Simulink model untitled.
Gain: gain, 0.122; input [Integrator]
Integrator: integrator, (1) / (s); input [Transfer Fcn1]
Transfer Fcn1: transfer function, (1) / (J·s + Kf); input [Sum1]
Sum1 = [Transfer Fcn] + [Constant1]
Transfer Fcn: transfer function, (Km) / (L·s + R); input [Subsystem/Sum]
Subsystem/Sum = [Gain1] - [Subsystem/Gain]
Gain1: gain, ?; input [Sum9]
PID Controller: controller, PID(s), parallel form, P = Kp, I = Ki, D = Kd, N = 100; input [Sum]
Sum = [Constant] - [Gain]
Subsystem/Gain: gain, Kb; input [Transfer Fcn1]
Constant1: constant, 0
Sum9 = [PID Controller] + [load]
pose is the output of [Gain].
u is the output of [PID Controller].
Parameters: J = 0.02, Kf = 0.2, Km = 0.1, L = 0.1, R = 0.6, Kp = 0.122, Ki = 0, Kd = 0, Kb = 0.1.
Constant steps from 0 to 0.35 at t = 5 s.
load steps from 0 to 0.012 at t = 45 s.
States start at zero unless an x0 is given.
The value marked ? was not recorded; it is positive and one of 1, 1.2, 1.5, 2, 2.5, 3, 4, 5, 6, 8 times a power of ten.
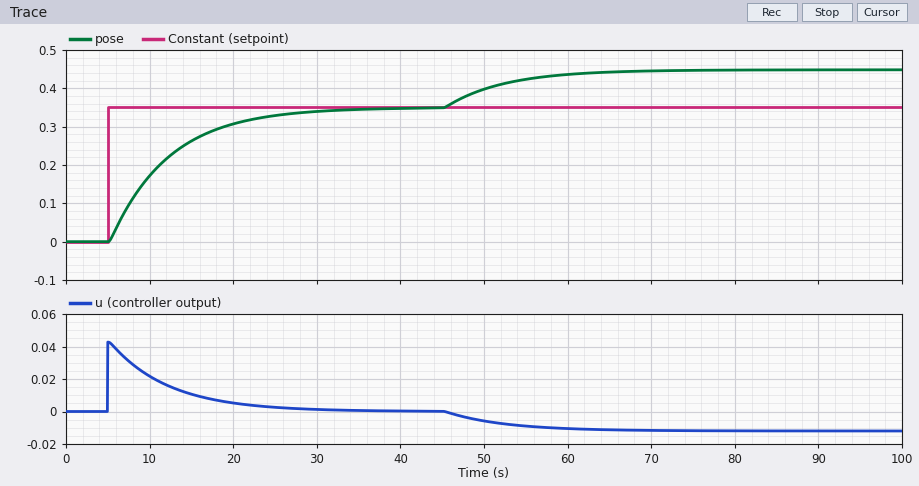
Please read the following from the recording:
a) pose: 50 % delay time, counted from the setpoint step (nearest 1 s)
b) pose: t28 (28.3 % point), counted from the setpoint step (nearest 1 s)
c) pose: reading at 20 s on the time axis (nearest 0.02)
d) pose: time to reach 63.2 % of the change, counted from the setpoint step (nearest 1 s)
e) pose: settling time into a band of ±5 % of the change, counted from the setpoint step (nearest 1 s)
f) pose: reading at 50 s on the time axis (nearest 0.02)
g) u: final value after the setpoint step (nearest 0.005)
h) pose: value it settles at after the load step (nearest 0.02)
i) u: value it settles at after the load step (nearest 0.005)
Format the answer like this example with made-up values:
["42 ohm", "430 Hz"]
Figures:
["5 s", "3 s", "0.30", "7 s", "21 s", "0.40", "0.000", "0.44", "-0.010"]
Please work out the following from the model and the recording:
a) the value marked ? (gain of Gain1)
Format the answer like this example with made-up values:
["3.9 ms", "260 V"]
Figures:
["12"]
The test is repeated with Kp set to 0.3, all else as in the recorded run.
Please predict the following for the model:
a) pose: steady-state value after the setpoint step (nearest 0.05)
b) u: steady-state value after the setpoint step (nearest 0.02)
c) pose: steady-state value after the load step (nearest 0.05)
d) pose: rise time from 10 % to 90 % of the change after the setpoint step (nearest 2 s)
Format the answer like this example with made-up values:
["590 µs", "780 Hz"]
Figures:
["0.35", "0.00", "0.40", "6 s"]
